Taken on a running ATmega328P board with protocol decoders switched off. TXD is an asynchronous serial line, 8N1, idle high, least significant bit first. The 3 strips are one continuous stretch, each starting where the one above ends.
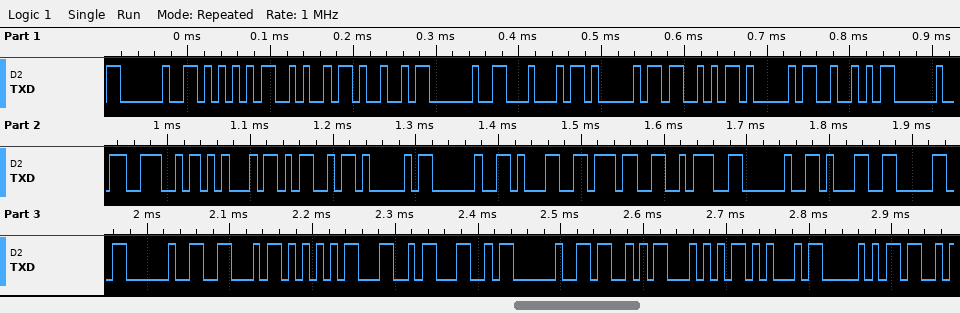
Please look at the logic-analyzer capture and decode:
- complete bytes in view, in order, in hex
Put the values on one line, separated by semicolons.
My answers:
20 55 4A 49 20 44 41 53 41 52 20 4E 45 4D 41 20 31 37 3A 20 31 30 20 46 55 4C 4C 20 53 54 45 50
